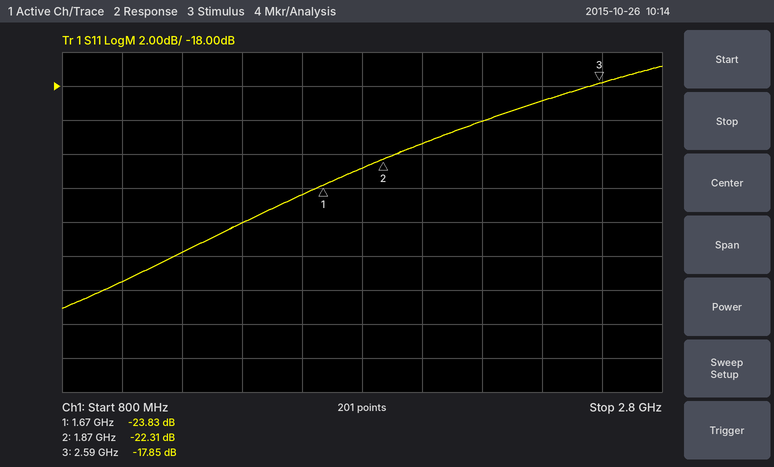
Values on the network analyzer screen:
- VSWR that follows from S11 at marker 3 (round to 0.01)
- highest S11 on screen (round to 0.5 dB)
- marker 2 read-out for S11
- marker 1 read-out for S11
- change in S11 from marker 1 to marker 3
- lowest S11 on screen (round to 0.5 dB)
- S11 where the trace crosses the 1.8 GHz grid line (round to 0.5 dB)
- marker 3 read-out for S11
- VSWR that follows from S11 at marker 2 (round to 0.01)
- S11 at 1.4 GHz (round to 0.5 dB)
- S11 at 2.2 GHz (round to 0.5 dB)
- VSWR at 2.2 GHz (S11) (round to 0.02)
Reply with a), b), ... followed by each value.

a) 1.29
b) -17.0 dB
c) -22.31 dB
d) -23.83 dB
e) 5.98 dB
f) -31.0 dB
g) -23.0 dB
h) -17.85 dB
i) 1.17
j) -26.0 dB
k) -20.0 dB
l) 1.22
